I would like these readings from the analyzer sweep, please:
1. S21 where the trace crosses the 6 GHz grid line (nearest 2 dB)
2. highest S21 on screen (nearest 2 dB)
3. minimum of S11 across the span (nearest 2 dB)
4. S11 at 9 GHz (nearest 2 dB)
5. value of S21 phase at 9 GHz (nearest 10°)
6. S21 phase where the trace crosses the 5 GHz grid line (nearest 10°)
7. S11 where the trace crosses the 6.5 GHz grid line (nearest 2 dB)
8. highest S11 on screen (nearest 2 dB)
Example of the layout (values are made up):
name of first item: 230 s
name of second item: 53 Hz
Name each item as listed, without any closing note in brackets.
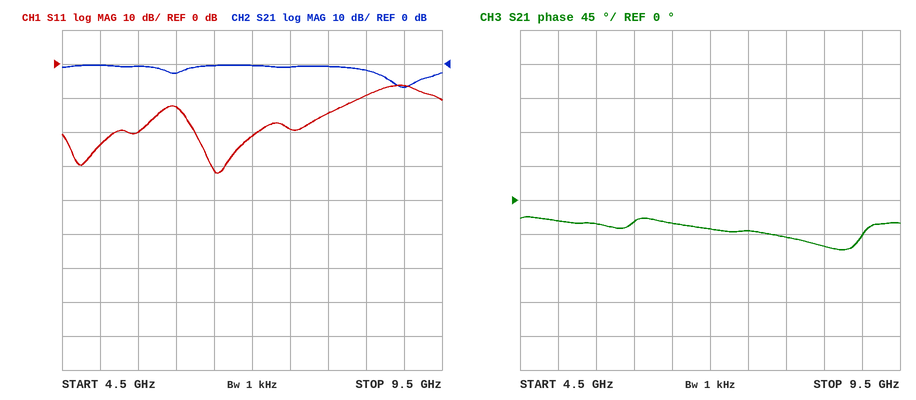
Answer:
S21 where the trace crosses the 6 GHz grid line: -2 dB
highest S21 on screen: 0 dB
minimum of S11 across the span: -32 dB
S11 at 9 GHz: -6 dB
value of S21 phase at 9 GHz: -50°
S21 phase where the trace crosses the 5 GHz grid line: -30°
S11 where the trace crosses the 6.5 GHz grid line: -32 dB
highest S11 on screen: -6 dB
